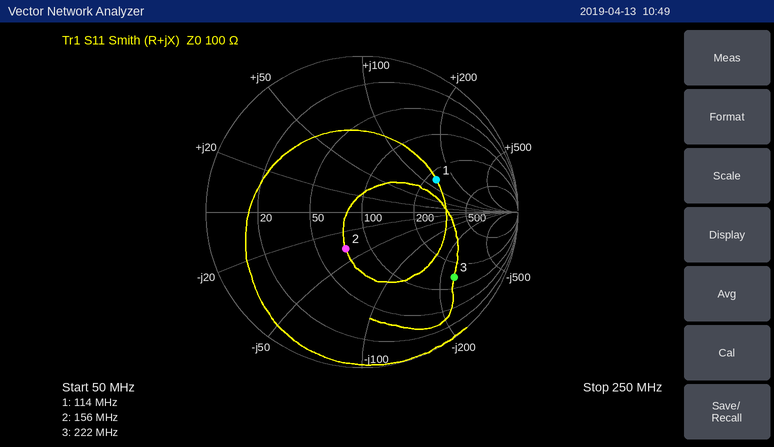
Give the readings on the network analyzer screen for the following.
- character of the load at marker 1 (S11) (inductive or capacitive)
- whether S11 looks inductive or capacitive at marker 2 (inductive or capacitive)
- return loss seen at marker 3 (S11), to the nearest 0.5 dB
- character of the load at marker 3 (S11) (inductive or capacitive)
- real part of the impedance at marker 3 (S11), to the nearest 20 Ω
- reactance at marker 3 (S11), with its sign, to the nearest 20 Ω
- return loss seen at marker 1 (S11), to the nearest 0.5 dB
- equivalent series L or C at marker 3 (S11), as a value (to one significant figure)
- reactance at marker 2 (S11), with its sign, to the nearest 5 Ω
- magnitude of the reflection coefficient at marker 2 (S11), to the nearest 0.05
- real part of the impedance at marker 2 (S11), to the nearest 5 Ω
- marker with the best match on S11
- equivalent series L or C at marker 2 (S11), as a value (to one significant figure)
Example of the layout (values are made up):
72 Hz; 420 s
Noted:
inductive; capacitive; 3.0 dB; capacitive; 140 Ω; -240 Ω; 5.5 dB; 3 pF; -35 Ω; 0.25; 75 Ω; marker 2; 30 pF
